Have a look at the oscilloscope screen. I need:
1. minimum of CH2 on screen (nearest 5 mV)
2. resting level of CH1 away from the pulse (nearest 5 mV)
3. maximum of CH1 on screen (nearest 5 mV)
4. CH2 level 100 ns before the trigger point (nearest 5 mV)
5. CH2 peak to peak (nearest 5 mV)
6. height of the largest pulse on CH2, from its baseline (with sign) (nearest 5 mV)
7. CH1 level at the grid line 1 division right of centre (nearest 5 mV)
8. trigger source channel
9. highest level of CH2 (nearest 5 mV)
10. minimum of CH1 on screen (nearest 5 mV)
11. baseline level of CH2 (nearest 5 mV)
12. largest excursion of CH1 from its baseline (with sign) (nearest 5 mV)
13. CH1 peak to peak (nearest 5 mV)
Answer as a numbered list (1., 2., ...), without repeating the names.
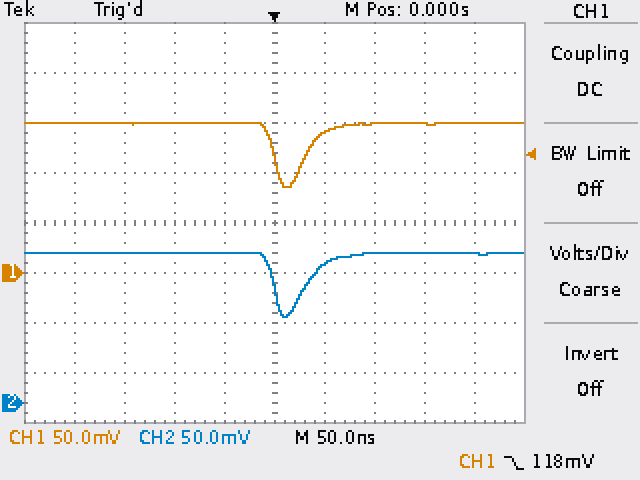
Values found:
1. 85 mV
2. 150 mV
3. 150 mV
4. 150 mV
5. 65 mV
6. -65 mV
7. 140 mV
8. CH1
9. 150 mV
10. 85 mV
11. 150 mV
12. -65 mV
13. 65 mV
